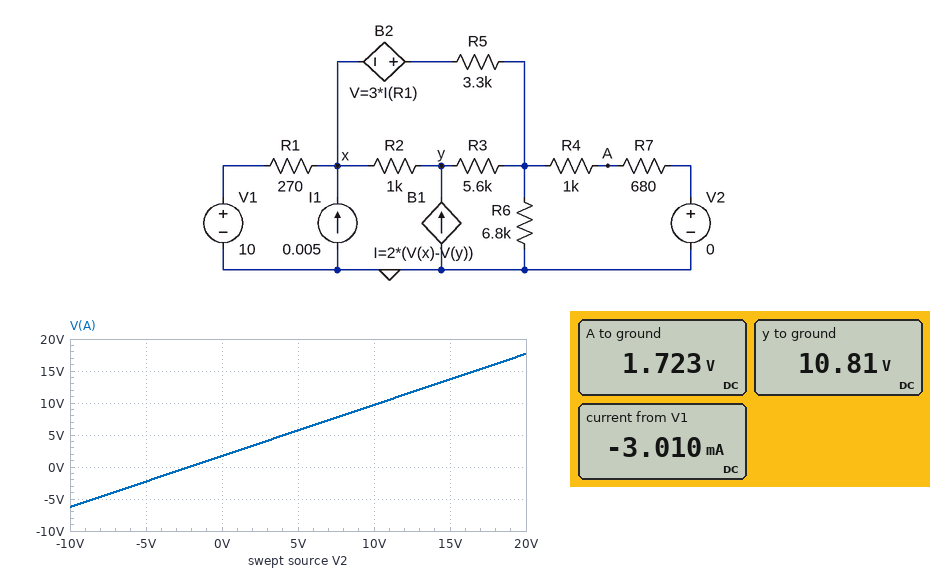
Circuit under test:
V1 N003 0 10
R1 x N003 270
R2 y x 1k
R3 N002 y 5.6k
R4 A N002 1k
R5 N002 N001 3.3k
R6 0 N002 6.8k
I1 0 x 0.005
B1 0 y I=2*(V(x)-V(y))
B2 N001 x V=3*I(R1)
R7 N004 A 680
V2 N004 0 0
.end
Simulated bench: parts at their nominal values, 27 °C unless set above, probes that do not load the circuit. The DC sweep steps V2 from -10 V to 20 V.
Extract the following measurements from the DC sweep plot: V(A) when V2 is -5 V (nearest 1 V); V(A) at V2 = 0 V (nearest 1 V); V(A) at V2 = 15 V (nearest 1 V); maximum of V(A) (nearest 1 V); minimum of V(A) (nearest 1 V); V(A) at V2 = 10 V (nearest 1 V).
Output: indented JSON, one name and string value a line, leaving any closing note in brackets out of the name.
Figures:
{
  "V(A) when V2 is -5 V": "-2 V",
  "V(A) at V2 = 0 V": "2 V",
  "V(A) at V2 = 15 V": "14 V",
  "maximum of V(A)": "18 V",
  "minimum of V(A)": "-6 V",
  "V(A) at V2 = 10 V": "10 V"
}
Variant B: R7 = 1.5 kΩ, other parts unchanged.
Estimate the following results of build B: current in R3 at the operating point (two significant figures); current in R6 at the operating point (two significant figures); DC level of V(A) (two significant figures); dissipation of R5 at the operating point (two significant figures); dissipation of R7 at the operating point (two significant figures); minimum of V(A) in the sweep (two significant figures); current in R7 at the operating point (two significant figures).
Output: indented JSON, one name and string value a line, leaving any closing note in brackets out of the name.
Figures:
{
  "current in R3 at the operating point": "1.0 mA",
  "current in R6 at the operating point": "750 µA",
  "DC level of V(A)": "3.1 V",
  "dissipation of R5 at the operating point": "10 mW",
  "dissipation of R7 at the operating point": "6.2 mW",
  "minimum of V(A) in the sweep": "-3.4 V",
  "current in R7 at the operating point": "2.0 mA"
}
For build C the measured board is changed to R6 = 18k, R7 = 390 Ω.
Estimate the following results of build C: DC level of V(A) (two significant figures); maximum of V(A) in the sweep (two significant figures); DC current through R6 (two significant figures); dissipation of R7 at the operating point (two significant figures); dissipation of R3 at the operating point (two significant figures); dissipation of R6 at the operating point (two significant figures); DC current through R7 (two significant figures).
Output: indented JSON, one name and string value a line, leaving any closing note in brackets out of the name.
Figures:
{
  "DC level of V(A)": "1.2 V",
  "maximum of V(A) in the sweep": "19 V",
  "DC current through R6": "230 µA",
  "dissipation of R7 at the operating point": "3.5 mW",
  "dissipation of R3 at the operating point": "7.9 mW",
  "dissipation of R6 at the operating point": "950 µW",
  "DC current through R7": "3.0 mA"
}
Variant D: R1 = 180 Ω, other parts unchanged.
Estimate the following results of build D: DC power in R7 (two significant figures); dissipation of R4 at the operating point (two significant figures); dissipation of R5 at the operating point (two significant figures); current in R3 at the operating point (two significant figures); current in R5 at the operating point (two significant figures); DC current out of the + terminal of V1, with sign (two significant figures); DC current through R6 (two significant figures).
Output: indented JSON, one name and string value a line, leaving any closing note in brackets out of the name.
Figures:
{
  "DC power in R7": "4.2 mW",
  "dissipation of R4 at the operating point": "6.1 mW",
  "dissipation of R5 at the operating point": "12 mW",
  "current in R3 at the operating point": "1.1 mA",
  "current in R5 at the operating point": "1.9 mA",
  "DC current out of the + terminal of V1, with sign": "-3.1 mA",
  "DC current through R6": "610 µA"
}
